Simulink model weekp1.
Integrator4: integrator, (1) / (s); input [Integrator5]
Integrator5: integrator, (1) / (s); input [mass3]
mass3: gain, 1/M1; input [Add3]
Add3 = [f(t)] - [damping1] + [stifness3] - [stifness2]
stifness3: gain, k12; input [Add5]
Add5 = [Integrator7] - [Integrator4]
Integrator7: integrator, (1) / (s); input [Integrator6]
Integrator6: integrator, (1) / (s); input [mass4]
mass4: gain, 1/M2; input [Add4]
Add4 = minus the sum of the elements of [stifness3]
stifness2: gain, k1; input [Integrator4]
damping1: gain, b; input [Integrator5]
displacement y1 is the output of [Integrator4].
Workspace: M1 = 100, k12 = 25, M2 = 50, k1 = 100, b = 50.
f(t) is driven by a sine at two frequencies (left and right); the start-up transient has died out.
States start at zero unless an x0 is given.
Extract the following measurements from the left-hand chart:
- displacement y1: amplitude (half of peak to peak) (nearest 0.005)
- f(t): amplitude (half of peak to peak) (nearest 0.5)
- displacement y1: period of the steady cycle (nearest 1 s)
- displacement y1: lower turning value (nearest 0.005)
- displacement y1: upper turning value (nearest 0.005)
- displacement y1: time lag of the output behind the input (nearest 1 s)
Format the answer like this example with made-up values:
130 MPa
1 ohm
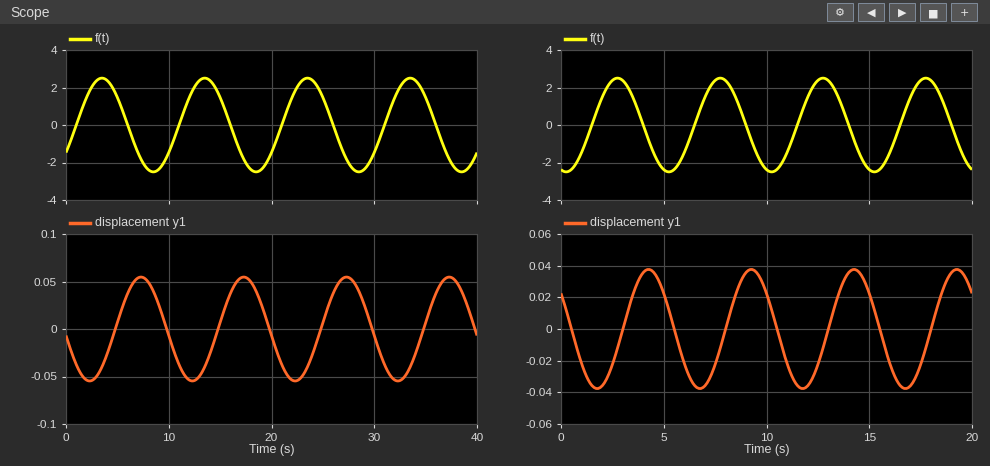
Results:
0.055
2.5
10 s
-0.055
0.055
4 s
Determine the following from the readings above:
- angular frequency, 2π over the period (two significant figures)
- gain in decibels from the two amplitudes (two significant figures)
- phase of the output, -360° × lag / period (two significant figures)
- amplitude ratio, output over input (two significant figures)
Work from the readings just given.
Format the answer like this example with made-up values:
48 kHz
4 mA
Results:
0.63 rad/s
-33 dB
-140°
0.022
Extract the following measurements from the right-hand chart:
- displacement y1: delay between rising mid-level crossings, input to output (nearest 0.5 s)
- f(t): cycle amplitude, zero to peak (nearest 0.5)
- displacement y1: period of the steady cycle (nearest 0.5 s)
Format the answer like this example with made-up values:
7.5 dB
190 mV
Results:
1.5 s
2.5
5.0 s
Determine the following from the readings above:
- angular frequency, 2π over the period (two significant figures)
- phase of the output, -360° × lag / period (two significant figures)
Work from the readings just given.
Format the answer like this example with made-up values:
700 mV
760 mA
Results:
1.3 rad/s
-110°
